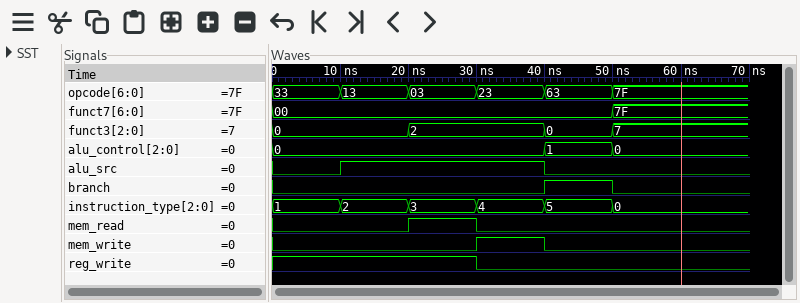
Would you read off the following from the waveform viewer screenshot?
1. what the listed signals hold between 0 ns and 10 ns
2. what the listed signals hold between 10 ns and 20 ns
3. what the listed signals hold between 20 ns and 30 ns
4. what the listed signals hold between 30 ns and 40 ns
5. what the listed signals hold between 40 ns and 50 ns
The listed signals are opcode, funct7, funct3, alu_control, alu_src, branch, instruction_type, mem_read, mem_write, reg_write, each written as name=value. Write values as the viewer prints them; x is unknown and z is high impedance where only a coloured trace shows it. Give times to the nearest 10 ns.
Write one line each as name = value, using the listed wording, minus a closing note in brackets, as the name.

what the listed signals hold between 0 ns and 10 ns = opcode=33, funct7=00, funct3=0, alu_control=0, alu_src=0, branch=0, instruction_type=1, mem_read=0, mem_write=0, reg_write=1
what the listed signals hold between 10 ns and 20 ns = opcode=13, funct7=00, funct3=0, alu_control=0, alu_src=1, branch=0, instruction_type=2, mem_read=0, mem_write=0, reg_write=1
what the listed signals hold between 20 ns and 30 ns = opcode=03, funct7=00, funct3=2, alu_control=0, alu_src=1, branch=0, instruction_type=3, mem_read=1, mem_write=0, reg_write=1
what the listed signals hold between 30 ns and 40 ns = opcode=23, funct7=00, funct3=2, alu_control=0, alu_src=1, branch=0, instruction_type=4, mem_read=0, mem_write=1, reg_write=0
what the listed signals hold between 40 ns and 50 ns = opcode=63, funct7=00, funct3=0, alu_control=1, alu_src=0, branch=1, instruction_type=5, mem_read=0, mem_write=0, reg_write=0
